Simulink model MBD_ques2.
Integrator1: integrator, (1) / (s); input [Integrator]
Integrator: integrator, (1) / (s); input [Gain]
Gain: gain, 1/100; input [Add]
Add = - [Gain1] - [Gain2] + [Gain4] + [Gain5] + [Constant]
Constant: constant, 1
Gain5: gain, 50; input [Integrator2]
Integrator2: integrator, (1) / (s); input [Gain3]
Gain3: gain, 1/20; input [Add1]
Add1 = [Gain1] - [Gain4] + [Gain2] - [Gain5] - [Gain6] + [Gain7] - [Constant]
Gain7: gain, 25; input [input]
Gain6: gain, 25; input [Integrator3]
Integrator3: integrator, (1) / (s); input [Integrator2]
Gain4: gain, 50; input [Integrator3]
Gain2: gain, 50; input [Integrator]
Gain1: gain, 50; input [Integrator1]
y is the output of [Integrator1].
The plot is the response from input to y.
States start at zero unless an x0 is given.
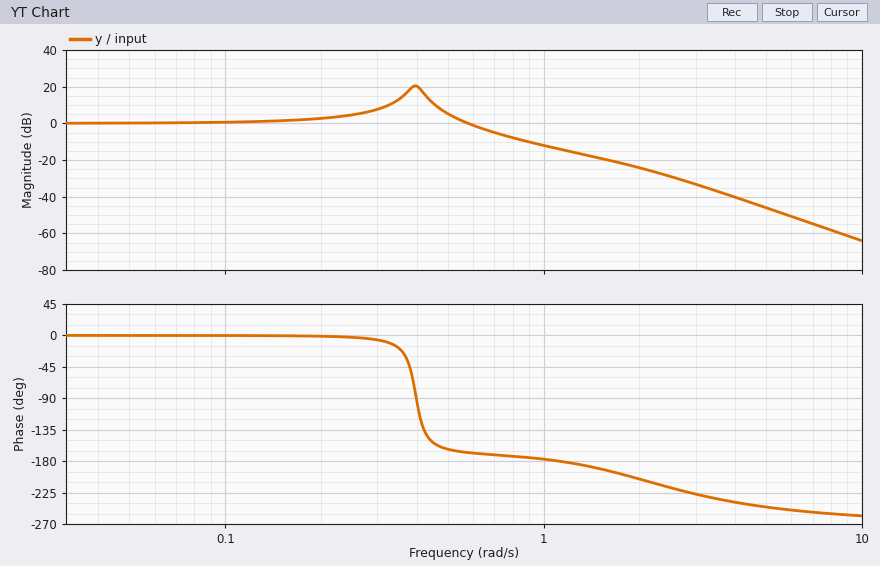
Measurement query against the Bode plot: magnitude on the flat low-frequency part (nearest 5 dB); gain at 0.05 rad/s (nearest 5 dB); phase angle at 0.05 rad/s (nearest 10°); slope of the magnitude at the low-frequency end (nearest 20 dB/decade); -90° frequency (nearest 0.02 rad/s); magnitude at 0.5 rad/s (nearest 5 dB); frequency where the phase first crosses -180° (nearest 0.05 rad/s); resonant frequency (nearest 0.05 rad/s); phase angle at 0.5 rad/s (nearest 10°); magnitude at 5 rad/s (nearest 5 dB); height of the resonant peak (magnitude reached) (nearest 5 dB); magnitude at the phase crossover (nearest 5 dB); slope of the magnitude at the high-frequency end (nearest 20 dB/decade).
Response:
0 dB
0 dB
0°
0 dB/decade
0.40 rad/s
5 dB
1.10 rad/s
0.40 rad/s
-160°
-45 dB
20 dB
-15 dB
-60 dB/decade
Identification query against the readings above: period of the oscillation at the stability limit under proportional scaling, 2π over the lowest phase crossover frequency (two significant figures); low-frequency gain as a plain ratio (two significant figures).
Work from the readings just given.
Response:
5.7 s
1.0
